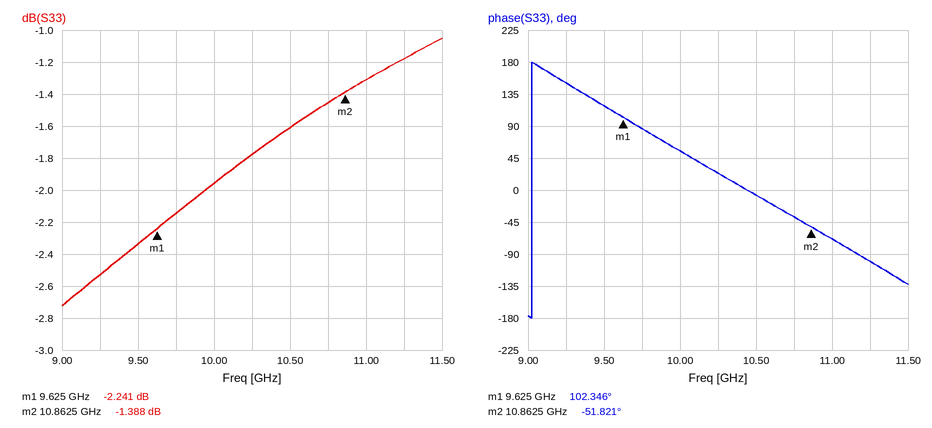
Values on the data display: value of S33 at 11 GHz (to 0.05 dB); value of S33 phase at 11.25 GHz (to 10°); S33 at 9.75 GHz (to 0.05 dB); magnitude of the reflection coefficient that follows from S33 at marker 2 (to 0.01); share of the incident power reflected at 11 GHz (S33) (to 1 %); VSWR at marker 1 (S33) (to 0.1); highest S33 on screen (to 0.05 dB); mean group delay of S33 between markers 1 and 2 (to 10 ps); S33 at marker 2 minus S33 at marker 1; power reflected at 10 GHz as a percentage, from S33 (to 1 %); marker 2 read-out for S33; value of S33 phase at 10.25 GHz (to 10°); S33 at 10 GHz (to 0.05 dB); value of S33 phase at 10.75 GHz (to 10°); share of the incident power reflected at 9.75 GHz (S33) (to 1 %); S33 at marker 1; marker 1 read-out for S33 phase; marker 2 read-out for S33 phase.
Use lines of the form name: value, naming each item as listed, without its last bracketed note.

value of S33 at 11 GHz: -1.30 dB
value of S33 phase at 11.25 GHz: -100°
S33 at 9.75 GHz: -2.15 dB
magnitude of the reflection coefficient that follows from S33 at marker 2: 0.85
share of the incident power reflected at 11 GHz (S33): 74 %
VSWR at marker 1 (S33): 7.8
highest S33 on screen: -1.05 dB
mean group delay of S33 between markers 1 and 2: 350 ps
S33 at marker 2 minus S33 at marker 1: 0.853 dB
power reflected at 10 GHz as a percentage, from S33: 64 %
marker 2 read-out for S33: -1.388 dB
value of S33 phase at 10.25 GHz: 20°
S33 at 10 GHz: -1.95 dB
value of S33 phase at 10.75 GHz: -40°
share of the incident power reflected at 9.75 GHz (S33): 61 %
S33 at marker 1: -2.241 dB
marker 1 read-out for S33 phase: 102.346°
marker 2 read-out for S33 phase: -51.821°
